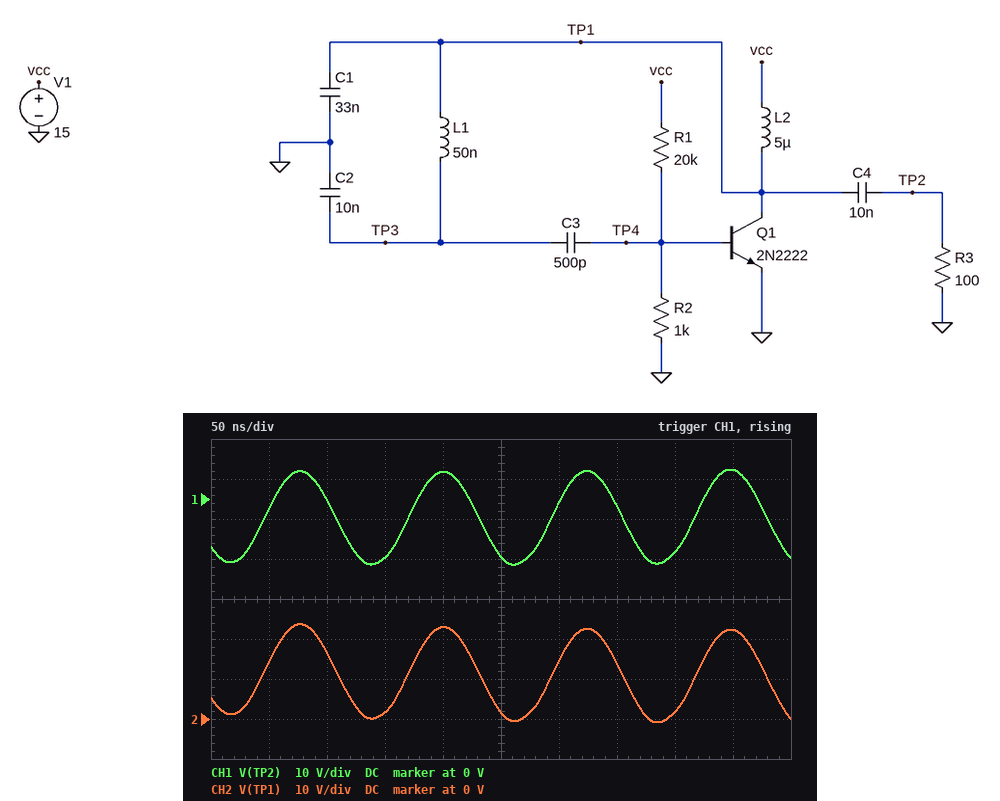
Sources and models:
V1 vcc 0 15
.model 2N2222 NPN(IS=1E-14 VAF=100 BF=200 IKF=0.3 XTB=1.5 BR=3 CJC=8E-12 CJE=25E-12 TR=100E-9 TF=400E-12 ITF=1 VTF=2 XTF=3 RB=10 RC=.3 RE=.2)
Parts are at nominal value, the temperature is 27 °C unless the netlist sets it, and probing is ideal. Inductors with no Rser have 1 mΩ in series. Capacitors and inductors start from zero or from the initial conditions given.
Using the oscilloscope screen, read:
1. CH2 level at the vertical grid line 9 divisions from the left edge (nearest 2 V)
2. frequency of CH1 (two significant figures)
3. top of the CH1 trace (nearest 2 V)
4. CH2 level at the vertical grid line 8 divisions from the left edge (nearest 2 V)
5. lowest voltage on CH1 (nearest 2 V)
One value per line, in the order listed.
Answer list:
22 V
8.1 MHz
8 V
2 V
-16 V
